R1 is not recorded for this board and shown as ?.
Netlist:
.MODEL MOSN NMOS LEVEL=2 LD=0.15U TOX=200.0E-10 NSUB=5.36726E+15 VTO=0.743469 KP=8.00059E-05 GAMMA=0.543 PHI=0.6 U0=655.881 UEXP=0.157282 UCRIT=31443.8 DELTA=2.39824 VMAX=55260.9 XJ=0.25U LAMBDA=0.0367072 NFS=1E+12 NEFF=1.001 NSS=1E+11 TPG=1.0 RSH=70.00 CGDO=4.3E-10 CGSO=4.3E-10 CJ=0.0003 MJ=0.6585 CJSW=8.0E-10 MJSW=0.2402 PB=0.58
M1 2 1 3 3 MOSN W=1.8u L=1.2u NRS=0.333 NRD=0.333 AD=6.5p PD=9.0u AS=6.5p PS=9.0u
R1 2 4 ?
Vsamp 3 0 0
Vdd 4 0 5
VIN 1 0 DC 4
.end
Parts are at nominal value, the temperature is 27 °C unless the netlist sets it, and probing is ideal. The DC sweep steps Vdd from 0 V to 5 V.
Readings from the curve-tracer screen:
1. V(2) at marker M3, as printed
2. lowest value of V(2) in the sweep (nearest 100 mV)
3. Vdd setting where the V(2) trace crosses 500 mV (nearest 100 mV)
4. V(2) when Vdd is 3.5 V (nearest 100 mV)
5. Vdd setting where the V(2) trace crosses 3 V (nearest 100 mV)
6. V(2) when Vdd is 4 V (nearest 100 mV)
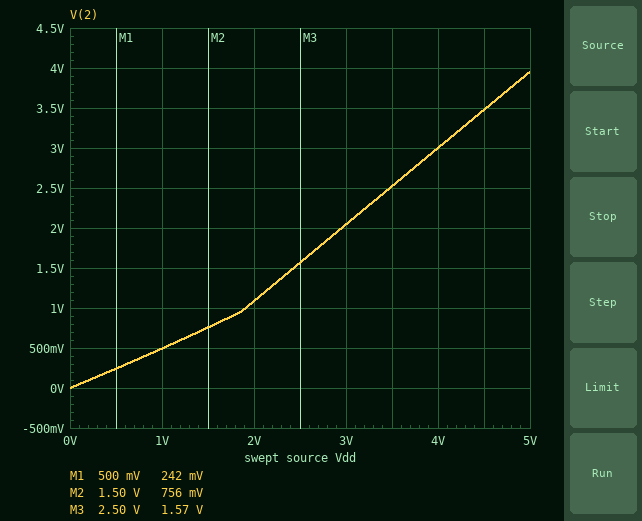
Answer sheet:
1.57 V
0 V
1.0 V
2.5 V
4.0 V
3.0 V
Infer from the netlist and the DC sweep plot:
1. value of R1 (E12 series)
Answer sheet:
3.3 kΩ
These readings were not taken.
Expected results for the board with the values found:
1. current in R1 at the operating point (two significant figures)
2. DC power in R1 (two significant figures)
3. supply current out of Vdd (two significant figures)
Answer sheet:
320 µA
330 µW
320 µA
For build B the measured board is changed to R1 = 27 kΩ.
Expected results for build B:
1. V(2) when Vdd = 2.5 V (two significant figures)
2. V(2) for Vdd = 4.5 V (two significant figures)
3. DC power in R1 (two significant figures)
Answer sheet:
260 mV
480 mV
740 µW
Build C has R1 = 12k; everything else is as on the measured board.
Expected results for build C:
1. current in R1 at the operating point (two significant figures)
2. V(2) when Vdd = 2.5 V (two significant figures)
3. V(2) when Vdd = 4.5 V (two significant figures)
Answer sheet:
280 µA
530 mV
1.2 V
